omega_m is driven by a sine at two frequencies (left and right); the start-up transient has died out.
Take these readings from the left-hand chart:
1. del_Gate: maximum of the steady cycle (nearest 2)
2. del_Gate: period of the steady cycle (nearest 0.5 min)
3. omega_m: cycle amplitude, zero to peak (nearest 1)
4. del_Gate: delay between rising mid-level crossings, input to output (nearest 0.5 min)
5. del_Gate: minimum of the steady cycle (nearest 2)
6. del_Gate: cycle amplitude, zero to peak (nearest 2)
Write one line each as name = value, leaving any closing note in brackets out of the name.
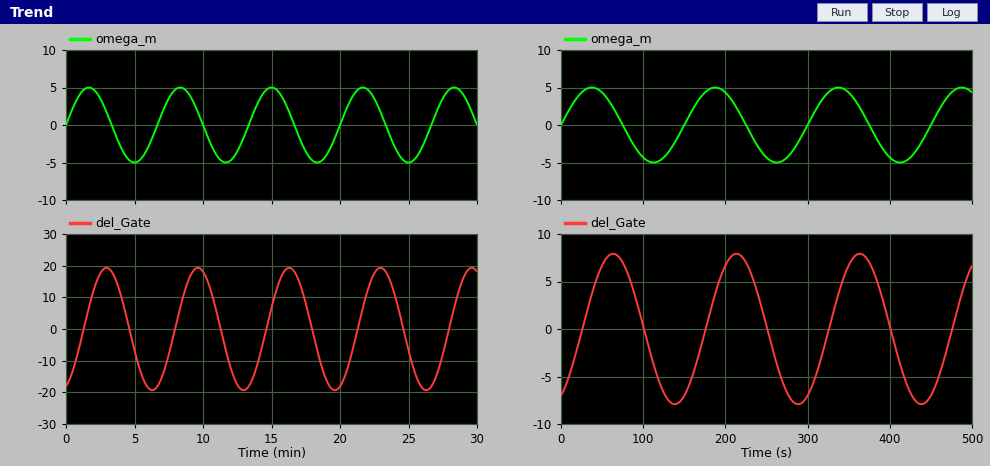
del_Gate: maximum of the steady cycle = 20
del_Gate: period of the steady cycle = 6.5 min
omega_m: cycle amplitude, zero to peak = 5
del_Gate: delay between rising mid-level crossings, input to output = 1.5 min
del_Gate: minimum of the steady cycle = -20
del_Gate: cycle amplitude, zero to peak = 20
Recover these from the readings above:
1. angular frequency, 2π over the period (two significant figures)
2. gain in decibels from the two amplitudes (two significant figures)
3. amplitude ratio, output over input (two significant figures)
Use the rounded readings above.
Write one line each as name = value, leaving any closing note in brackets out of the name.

angular frequency, 2π over the period = 0.97 rad/min
gain in decibels from the two amplitudes = 12 dB
amplitude ratio, output over input = 4.0
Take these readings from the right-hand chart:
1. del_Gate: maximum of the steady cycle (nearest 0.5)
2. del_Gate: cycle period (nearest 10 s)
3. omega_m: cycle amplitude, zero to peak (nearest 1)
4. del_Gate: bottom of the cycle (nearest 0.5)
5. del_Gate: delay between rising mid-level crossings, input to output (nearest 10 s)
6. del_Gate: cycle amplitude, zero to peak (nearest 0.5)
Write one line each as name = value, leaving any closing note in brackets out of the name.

del_Gate: maximum of the steady cycle = 8.0
del_Gate: cycle period = 150 s
omega_m: cycle amplitude, zero to peak = 5
del_Gate: bottom of the cycle = -8.0
del_Gate: delay between rising mid-level crossings, input to output = 30 s
del_Gate: cycle amplitude, zero to peak = 8.0
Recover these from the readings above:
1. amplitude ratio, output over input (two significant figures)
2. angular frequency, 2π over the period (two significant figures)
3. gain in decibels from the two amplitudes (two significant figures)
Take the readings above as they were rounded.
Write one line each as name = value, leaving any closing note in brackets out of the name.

amplitude ratio, output over input = 1.6
angular frequency, 2π over the period = 0.042 rad/s
gain in decibels from the two amplitudes = 4.1 dB
